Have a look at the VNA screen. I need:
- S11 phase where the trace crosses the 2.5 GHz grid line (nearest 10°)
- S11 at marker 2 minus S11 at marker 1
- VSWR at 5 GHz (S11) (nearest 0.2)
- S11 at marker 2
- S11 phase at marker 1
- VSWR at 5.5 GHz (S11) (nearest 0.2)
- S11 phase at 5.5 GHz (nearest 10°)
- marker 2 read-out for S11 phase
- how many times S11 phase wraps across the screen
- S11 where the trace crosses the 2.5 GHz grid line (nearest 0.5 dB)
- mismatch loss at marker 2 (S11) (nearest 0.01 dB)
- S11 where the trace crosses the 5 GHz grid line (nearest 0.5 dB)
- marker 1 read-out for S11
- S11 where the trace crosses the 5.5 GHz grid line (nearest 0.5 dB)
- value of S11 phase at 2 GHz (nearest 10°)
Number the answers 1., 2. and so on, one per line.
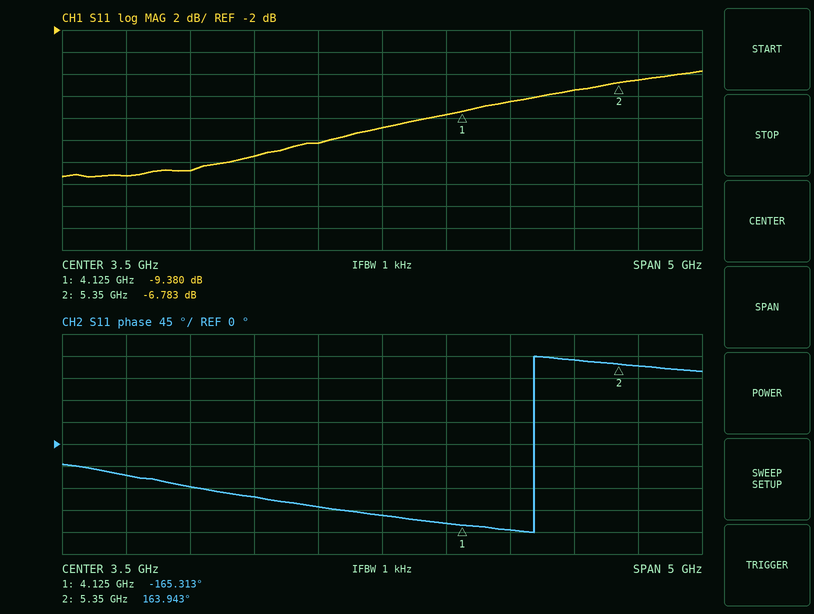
1. -110°
2. 2.597 dB
3. 2.4
4. -6.783 dB
5. -165.313°
6. 2.8
7. 160°
8. 163.943°
9. 1
10. -13.5 dB
11. 1.02 dB
12. -7.5 dB
13. -9.380 dB
14. -6.5 dB
15. -90°
